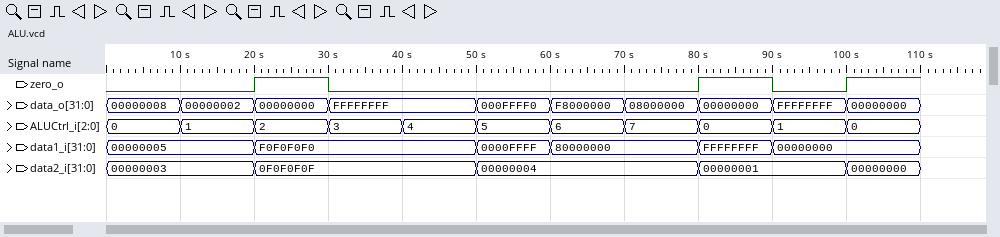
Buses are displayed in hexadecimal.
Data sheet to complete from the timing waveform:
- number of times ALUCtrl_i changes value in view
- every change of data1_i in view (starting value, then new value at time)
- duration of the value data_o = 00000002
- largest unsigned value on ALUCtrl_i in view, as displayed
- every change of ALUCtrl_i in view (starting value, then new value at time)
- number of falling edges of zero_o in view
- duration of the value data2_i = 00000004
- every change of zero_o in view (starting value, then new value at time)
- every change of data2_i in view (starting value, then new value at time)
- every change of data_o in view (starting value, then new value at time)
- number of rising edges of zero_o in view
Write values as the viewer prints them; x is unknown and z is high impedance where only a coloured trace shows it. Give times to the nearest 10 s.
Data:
10
00000005, F0F0F0F0 at 20 s, 0000FFFF at 50 s, 80000000 at 60 s, FFFFFFFF at 80 s, 00000000 at 90 s
10 s
7
0, 1 at 10 s, 2 at 20 s, 3 at 30 s, 4 at 40 s, 5 at 50 s, 6 at 60 s, 7 at 70 s, 0 at 80 s, 1 at 90 s, 0 at 100 s
2
30 s
0, 1 at 20 s, 0 at 30 s, 1 at 80 s, 0 at 90 s, 1 at 100 s
00000003, 0F0F0F0F at 20 s, 00000004 at 50 s, 00000001 at 80 s, 00000000 at 100 s
00000008, 00000002 at 10 s, 00000000 at 20 s, FFFFFFFF at 30 s, 000FFFF0 at 50 s, F8000000 at 60 s, 08000000 at 70 s, 00000000 at 80 s, FFFFFFFF at 90 s, 00000000 at 100 s
3
